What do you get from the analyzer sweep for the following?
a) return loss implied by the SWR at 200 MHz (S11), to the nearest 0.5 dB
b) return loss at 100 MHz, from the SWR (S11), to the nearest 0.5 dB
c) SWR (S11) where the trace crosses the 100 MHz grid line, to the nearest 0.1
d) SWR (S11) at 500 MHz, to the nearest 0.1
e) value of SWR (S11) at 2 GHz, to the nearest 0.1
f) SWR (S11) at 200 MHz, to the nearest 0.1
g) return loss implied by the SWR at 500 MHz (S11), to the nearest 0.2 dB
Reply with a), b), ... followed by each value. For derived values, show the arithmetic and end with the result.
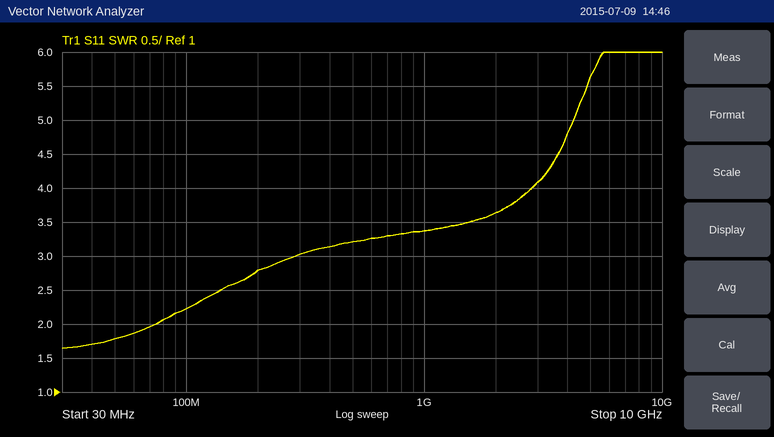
a) −20 log10((2.8 − 1)/(2.8 + 1)) ≈ 6.5 dB
b) −20 log10((2.2 − 1)/(2.2 + 1)) ≈ 8.5 dB
c) 2.2
d) 3.2
e) 3.6
f) 2.8
g) −20 log10((3.2 − 1)/(3.2 + 1)) ≈ 5.6 dB
